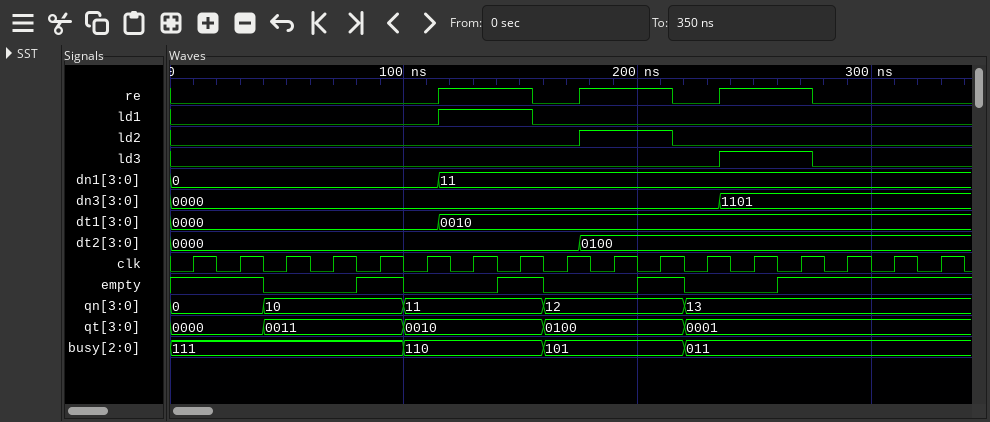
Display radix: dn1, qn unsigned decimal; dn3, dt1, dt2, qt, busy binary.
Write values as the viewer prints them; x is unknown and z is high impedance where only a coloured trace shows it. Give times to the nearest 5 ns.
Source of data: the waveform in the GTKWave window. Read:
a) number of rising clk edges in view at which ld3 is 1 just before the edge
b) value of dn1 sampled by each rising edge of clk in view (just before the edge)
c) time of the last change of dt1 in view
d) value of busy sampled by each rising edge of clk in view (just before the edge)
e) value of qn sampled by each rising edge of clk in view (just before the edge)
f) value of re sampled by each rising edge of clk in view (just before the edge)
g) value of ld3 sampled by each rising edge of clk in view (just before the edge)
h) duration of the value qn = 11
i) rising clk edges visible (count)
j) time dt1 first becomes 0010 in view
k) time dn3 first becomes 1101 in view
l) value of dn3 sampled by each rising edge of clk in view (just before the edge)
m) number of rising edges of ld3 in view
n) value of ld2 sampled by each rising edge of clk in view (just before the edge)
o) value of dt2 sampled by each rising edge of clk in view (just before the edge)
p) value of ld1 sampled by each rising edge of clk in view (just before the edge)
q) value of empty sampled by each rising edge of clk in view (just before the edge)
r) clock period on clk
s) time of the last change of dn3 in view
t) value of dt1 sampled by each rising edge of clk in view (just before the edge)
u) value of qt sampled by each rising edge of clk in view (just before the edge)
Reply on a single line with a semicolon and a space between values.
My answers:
2; 0, 0, 0, 0, 0, 0, 11, 11, 11, 11, 11, 11, 11, 11, 11, 11, 11; 115 ns; 111, 111, 111, 111, 111, 110, 110, 110, 101, 101, 101, 011, 011, 011, 011, 011, 011; 0, 0, 10, 10, 10, 11, 11, 11, 12, 12, 12, 13, 13, 13, 13, 13, 13; 0 0 0 0 0 0 1 1 0 1 1 0 1 1 0 0 0; 0 0 0 0 0 0 0 0 0 0 0 0 1 1 0 0 0; 60 ns; 17; 115 ns; 235 ns; 0000, 0000, 0000, 0000, 0000, 0000, 0000, 0000, 0000, 0000, 0000, 0000, 1101, 1101, 1101, 1101, 1101; 1; 0 0 0 0 0 0 0 0 0 1 1 0 0 0 0 0 0; 0000, 0000, 0000, 0000, 0000, 0000, 0000, 0000, 0000, 0100, 0100, 0100, 0100, 0100, 0100, 0100, 0100; 0 0 0 0 0 0 1 1 0 0 0 0 0 0 0 0 0; 1 1 0 0 1 0 0 1 0 0 1 0 0 1 1 1 1; 20 ns; 235 ns; 0000, 0000, 0000, 0000, 0000, 0000, 0010, 0010, 0010, 0010, 0010, 0010, 0010, 0010, 0010, 0010, 0010; 0000, 0000, 0011, 0011, 0011, 0010, 0010, 0010, 0100, 0100, 0100, 0001, 0001, 0001, 0001, 0001, 0001
